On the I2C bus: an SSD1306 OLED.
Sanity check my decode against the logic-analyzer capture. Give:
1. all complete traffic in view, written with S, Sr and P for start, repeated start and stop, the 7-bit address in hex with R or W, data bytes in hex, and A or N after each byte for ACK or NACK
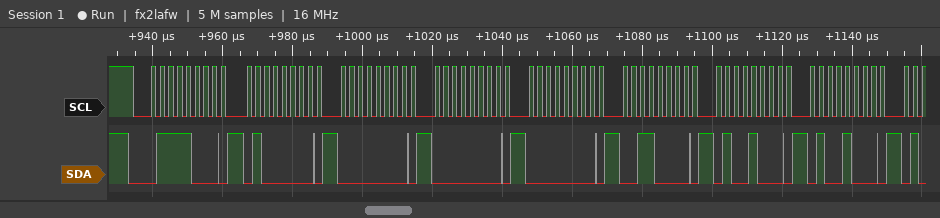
S 3CW A 40 A 00 A 00 A 00 A 30 A 48 A 48 A
